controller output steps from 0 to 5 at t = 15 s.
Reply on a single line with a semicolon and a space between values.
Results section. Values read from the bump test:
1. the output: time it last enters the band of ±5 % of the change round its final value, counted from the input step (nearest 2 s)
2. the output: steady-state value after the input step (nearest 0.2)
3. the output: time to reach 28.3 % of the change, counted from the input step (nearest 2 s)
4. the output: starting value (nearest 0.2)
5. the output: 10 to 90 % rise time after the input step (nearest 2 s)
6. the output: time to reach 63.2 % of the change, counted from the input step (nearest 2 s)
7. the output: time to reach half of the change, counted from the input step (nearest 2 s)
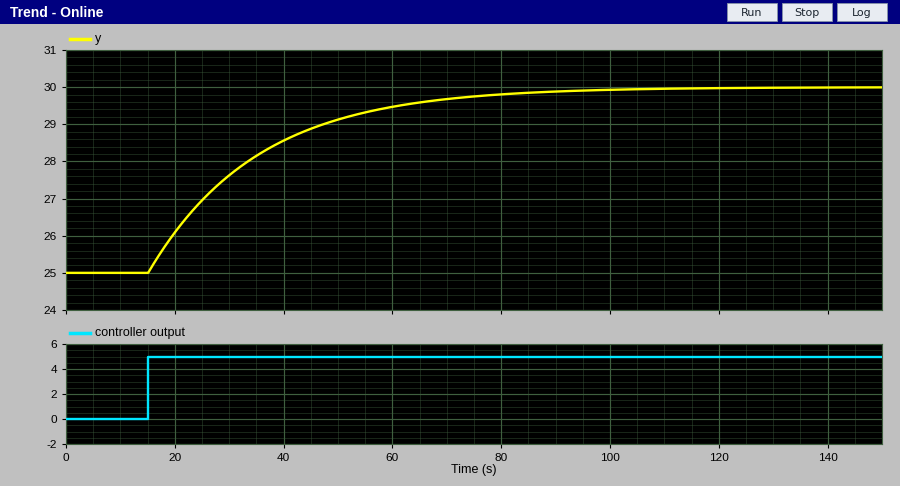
60 s; 30.0; 6 s; 25.0; 44 s; 20 s; 14 s
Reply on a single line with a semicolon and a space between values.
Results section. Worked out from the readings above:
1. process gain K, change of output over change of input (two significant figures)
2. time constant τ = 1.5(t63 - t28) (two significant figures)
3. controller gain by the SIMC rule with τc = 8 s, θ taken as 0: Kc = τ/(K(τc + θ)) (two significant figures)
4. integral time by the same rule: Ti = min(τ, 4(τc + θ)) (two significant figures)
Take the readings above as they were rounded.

1.0; 21 s; 2.6; 21 s
